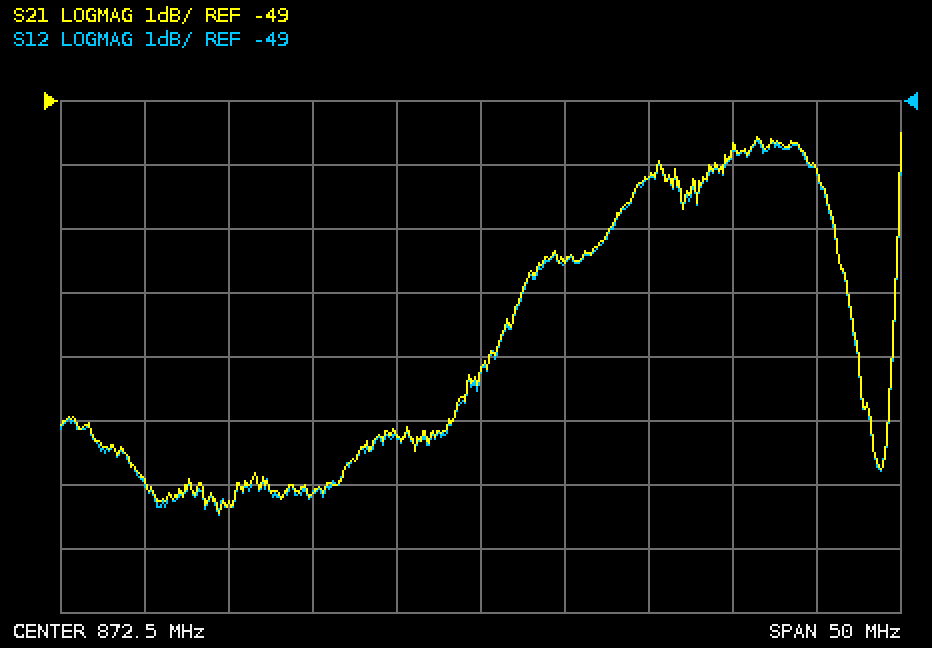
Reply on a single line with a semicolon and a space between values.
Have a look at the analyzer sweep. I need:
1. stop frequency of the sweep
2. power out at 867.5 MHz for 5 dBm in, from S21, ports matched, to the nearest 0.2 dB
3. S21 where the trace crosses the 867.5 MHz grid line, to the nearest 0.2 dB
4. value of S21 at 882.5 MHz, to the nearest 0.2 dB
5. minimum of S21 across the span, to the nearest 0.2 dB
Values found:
897.5 MHz; -49.2 dBm; -54.2 dB; -50.2 dB; -55.4 dB
